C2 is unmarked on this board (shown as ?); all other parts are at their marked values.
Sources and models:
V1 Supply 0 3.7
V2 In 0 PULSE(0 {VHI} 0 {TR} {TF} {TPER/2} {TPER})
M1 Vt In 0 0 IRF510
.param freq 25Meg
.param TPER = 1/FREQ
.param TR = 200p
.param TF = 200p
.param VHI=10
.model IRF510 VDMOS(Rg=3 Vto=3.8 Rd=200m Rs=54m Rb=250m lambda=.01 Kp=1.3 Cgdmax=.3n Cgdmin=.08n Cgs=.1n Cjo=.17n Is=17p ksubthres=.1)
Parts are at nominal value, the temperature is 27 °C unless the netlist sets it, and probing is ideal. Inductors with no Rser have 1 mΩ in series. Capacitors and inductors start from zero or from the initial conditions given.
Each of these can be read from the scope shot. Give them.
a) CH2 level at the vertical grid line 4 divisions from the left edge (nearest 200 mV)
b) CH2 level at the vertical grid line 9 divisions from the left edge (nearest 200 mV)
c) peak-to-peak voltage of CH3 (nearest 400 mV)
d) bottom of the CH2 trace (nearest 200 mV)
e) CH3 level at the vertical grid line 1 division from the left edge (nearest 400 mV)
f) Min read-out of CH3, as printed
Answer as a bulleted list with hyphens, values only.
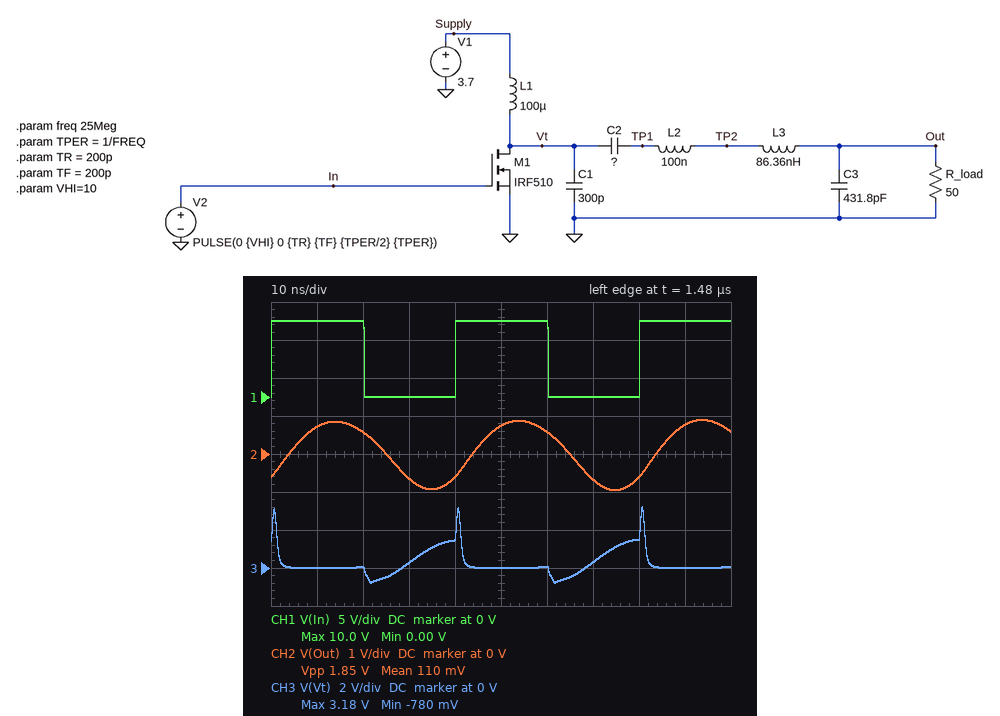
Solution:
- -600 mV
- 800 mV
- 4.0 V
- -1.0 V
- 0 V
- -780 mV
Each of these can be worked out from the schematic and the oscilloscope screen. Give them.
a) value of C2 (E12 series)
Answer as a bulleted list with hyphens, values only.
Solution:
- 1.2 nF
